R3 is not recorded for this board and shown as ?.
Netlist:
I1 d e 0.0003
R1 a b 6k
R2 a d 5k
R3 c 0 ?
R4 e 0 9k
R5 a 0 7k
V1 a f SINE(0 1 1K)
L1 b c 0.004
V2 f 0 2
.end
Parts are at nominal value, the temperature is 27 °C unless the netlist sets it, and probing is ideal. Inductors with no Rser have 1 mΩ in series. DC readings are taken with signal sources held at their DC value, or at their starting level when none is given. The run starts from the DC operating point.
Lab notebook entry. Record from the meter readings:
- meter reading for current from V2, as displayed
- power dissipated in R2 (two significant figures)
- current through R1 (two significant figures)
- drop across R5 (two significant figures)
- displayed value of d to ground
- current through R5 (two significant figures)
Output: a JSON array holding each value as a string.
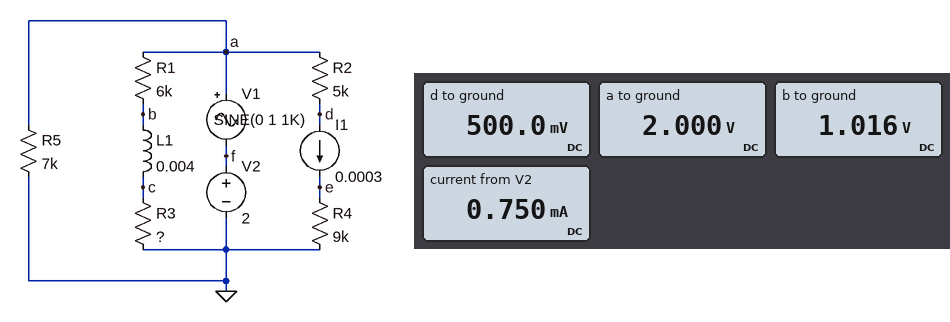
["0.750 mA", "450 µW", "160 µA", "2.0 V", "500.0 mV", "290 µA"]
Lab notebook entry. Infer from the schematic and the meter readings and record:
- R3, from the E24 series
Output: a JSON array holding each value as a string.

["6.2 kΩ"]
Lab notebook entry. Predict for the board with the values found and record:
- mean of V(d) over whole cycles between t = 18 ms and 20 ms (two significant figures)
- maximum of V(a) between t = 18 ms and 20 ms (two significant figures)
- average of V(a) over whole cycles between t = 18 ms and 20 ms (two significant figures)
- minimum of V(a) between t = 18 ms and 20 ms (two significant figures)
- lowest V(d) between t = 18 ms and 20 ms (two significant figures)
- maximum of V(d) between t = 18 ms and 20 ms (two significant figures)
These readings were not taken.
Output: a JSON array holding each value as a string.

["500 mV", "3.0 V", "2.0 V", "1.0 V", "-500 mV", "1.5 V"]
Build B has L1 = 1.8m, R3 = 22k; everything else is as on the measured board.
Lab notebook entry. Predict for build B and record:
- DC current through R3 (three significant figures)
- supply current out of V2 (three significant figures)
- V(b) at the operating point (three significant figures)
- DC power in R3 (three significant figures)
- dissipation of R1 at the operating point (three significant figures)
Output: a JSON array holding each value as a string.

["71.4 µA", "657 µA", "1.57 V", "112 µW", "30.6 µW"]
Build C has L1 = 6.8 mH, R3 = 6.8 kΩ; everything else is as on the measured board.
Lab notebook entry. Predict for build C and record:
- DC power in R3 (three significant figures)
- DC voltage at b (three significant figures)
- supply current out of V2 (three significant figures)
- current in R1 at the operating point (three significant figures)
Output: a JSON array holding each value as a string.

["166 µW", "1.06 V", "742 µA", "156 µA"]
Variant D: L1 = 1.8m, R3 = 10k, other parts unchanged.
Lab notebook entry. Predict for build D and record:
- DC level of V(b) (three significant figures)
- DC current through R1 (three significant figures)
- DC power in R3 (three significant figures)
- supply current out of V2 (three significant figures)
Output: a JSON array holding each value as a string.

["1.25 V", "125 µA", "156 µW", "711 µA"]
